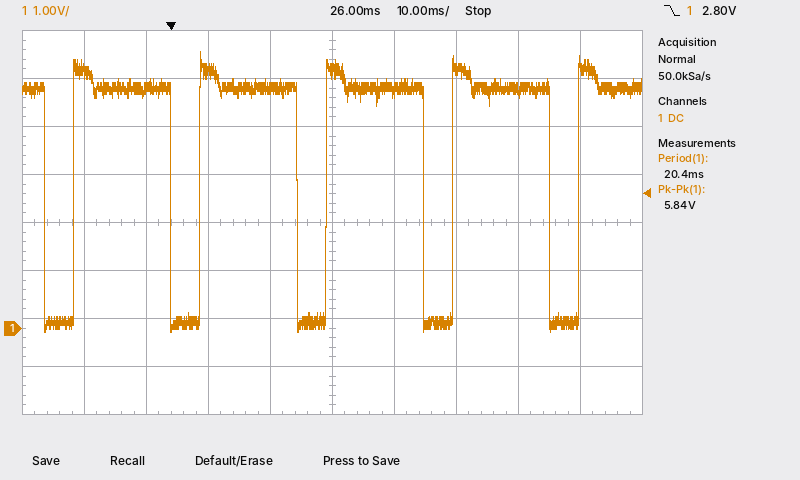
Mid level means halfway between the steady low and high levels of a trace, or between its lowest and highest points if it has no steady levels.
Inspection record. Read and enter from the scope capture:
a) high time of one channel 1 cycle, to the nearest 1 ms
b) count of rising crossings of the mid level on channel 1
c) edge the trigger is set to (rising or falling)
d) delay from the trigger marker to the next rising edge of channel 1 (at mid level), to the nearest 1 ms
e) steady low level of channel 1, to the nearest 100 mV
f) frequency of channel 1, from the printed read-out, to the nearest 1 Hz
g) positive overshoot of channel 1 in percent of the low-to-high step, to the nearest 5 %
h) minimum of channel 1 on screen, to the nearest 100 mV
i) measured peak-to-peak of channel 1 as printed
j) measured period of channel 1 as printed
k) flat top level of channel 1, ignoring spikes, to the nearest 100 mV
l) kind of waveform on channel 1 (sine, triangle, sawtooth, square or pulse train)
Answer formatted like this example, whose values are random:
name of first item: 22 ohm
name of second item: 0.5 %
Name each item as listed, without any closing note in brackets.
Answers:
high time of one channel 1 cycle, to the nearest 1 ms: 16 ms
count of rising crossings of the mid level on channel 1: 5
edge the trigger is set to: falling
delay from the trigger marker to the next rising edge of channel 1 (at mid level), to the nearest 1 ms: 5 ms
steady low level of channel 1, to the nearest 100 mV: 100 mV
frequency of channel 1, from the printed read-out, to the nearest 1 Hz: 49 Hz
positive overshoot of channel 1 in percent of the low-to-high step, to the nearest 5 %: 15 %
minimum of channel 1 on screen, to the nearest 100 mV: -100 mV
measured peak-to-peak of channel 1 as printed: 5.84 V
measured period of channel 1 as printed: 20.4 ms
flat top level of channel 1, ignoring spikes, to the nearest 100 mV: 5.0 V
kind of waveform on channel 1: pulse train
